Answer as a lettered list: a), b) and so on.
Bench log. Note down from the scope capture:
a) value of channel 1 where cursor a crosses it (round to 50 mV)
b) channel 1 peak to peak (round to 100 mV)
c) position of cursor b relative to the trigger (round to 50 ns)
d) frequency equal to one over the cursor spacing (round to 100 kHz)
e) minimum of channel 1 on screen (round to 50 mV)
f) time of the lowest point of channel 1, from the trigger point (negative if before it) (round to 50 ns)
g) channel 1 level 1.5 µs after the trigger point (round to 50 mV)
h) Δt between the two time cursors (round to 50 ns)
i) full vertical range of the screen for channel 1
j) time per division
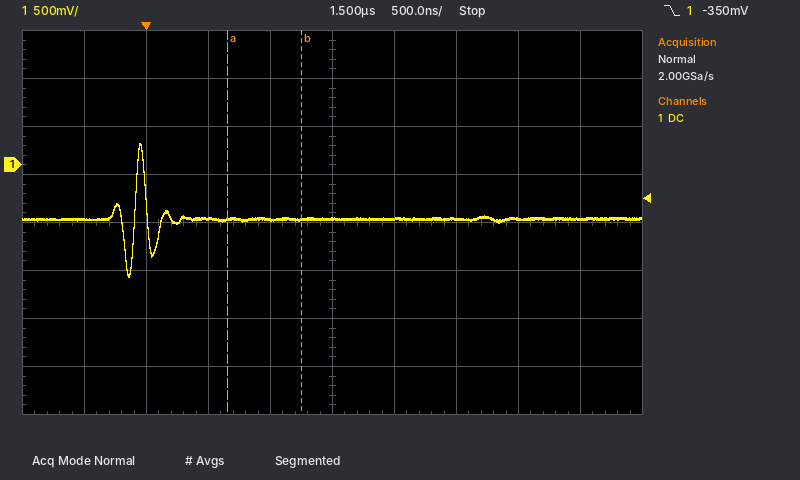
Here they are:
a) -550 mV
b) 1.40 V
c) +1.25 µs
d) 1.7 MHz
e) -1.15 V
f) -150 ns
g) -550 mV
h) 600 ns
i) 4 V
j) 500 ns
